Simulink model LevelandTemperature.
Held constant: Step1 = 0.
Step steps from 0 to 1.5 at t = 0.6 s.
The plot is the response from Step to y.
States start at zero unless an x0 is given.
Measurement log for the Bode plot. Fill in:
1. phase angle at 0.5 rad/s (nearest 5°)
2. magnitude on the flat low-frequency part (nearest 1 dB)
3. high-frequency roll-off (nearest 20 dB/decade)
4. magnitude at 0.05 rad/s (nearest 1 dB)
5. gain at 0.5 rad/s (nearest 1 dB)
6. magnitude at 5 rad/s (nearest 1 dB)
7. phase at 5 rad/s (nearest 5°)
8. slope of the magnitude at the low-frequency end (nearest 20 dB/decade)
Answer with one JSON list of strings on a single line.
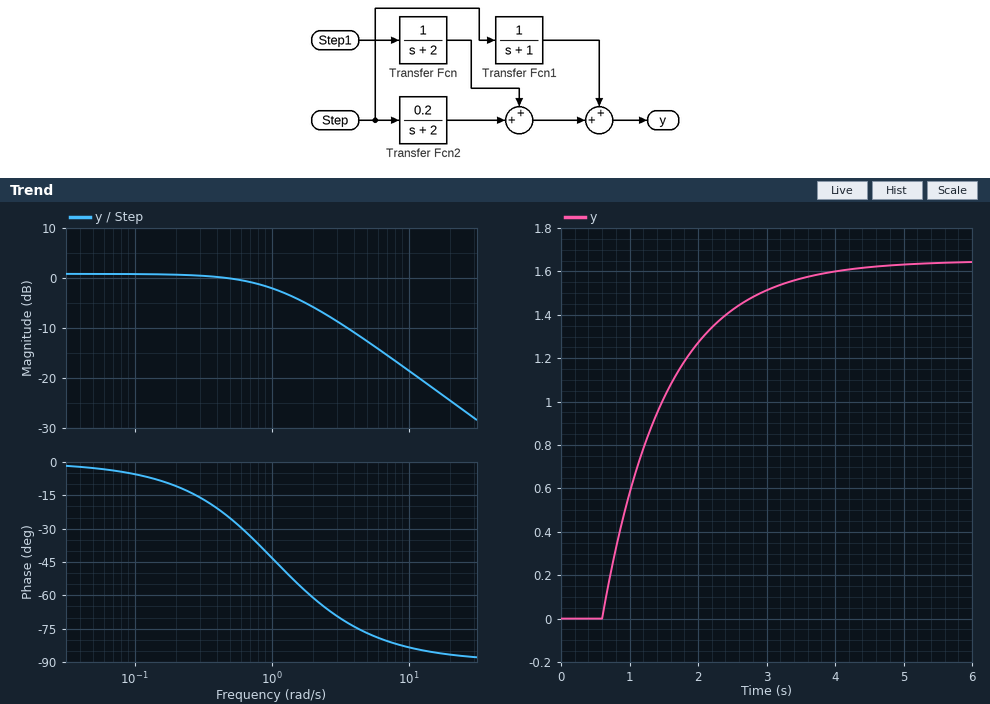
["-25°", "1 dB", "-20 dB/decade", "1 dB", "0 dB", "-13 dB", "-75°", "0 dB/decade"]
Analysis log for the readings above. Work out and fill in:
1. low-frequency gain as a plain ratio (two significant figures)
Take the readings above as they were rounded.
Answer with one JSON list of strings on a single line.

["1.1"]
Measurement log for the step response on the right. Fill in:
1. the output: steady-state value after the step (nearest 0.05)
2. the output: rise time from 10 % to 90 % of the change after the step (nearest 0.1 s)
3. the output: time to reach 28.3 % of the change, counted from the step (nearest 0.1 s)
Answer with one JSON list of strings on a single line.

["1.65", "2.1 s", "0.3 s"]
